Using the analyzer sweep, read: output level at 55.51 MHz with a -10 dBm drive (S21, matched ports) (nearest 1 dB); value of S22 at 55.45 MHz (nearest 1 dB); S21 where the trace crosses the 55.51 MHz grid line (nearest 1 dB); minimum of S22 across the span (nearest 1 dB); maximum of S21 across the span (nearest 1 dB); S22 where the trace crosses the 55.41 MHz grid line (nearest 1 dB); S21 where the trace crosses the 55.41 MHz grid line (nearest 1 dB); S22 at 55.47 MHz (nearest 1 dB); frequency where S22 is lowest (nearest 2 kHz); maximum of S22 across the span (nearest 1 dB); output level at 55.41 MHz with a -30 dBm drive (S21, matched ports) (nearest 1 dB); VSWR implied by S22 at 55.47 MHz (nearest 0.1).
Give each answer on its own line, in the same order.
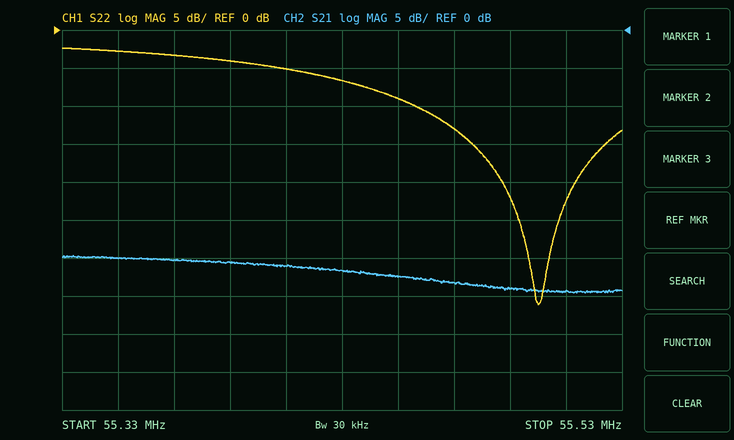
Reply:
-44 dBm
-9 dB
-34 dB
-36 dB
-30 dB
-5 dB
-31 dB
-13 dB
55.500 MHz
-2 dB
-61 dBm
1.6
